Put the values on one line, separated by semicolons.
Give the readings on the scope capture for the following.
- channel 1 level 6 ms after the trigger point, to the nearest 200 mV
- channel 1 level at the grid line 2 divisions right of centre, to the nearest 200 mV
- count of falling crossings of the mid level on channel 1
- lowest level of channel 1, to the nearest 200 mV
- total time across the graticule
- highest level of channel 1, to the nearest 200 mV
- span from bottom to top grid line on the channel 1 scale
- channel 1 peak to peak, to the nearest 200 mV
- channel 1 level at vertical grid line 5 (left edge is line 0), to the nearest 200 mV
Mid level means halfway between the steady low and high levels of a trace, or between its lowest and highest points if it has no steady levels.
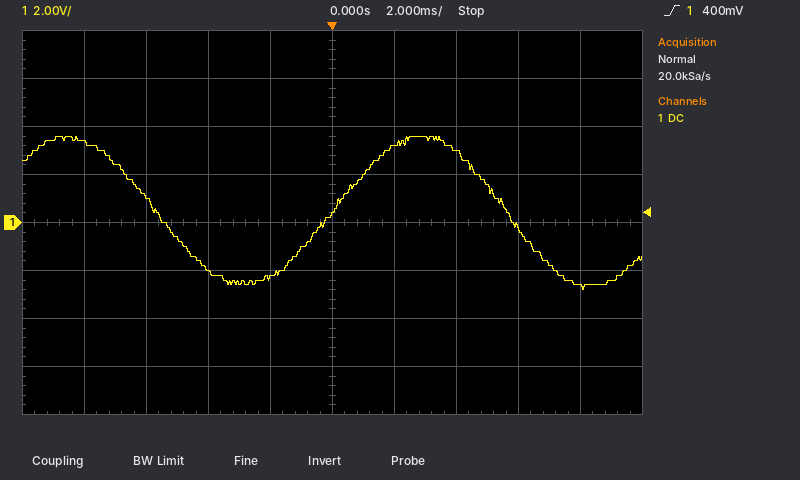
-200 mV; 3.0 V; 2; -2.8 V; 20 ms; 3.6 V; 16 V; 6.4 V; 400 mV
